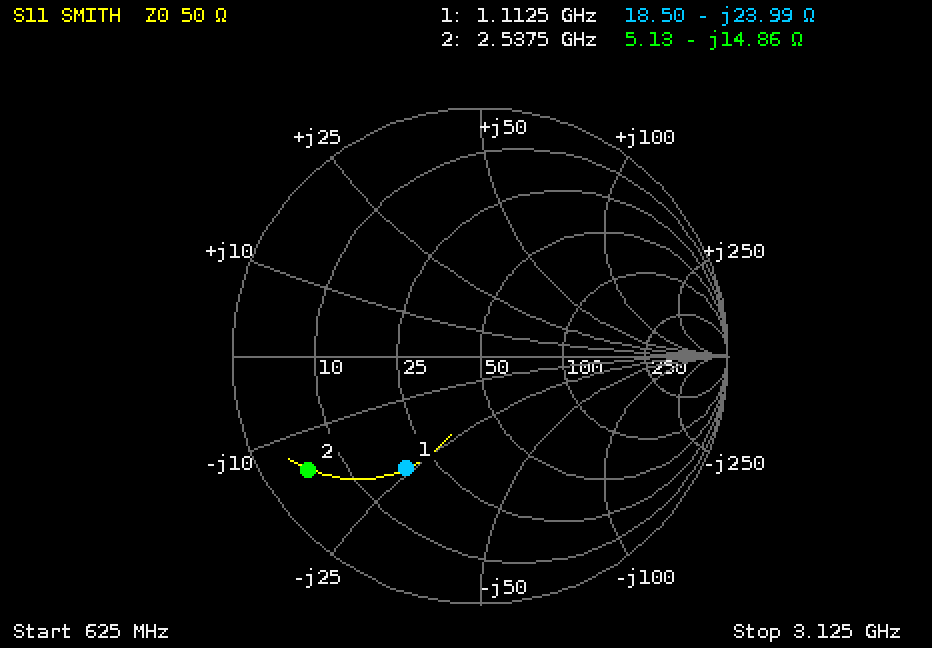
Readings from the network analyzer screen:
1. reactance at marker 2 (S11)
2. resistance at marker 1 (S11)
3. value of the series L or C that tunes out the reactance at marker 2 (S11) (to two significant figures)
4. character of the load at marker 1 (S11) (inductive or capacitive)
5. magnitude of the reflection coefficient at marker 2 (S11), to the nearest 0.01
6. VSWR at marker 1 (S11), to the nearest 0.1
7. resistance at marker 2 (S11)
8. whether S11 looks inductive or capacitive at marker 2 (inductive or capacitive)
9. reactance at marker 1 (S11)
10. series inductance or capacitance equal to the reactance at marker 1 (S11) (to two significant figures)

-14.86 Ω
18.50 Ω
930 pH
capacitive
0.83
3.4
5.13 Ω
capacitive
-23.99 Ω
6.0 pF
